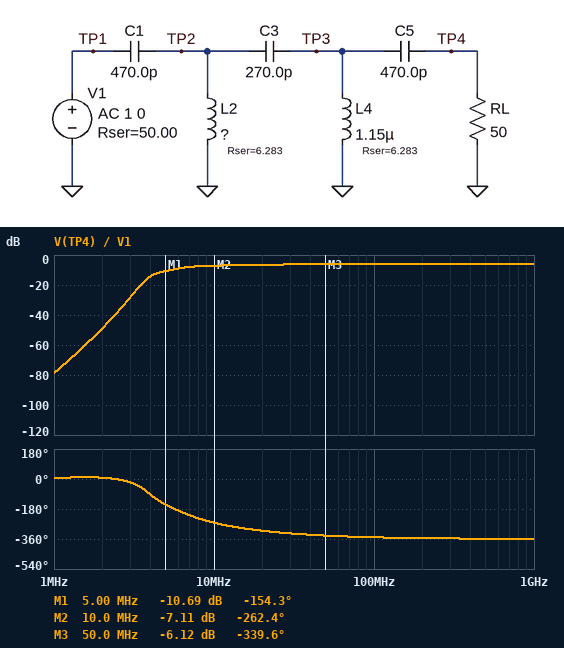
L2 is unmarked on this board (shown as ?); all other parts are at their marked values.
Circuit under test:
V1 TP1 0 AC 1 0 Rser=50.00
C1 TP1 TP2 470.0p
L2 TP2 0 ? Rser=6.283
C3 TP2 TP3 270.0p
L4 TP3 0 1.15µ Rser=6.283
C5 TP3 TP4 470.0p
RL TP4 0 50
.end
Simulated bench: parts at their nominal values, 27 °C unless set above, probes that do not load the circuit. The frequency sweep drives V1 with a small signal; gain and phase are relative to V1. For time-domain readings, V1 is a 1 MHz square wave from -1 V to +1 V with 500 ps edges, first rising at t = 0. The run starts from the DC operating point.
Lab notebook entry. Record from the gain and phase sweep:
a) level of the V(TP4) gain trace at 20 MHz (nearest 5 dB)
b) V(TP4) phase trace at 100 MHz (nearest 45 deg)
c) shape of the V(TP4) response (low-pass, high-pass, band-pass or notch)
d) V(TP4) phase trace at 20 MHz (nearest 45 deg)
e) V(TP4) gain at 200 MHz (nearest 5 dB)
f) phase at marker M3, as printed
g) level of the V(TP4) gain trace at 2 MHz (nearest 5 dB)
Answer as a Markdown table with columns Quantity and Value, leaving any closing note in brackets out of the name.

| Quantity | Value |
|---|---|
| level of the V(TP4) gain trace at 20 MHz | -5 dB |
| V(TP4) phase trace at 100 MHz | -360 deg |
| shape of the V(TP4) response | high-pass |
| V(TP4) phase trace at 20 MHz | -315 deg |
| V(TP4) gain at 200 MHz | -5 dB |
| phase at marker M3, as printed | -339.6 deg |
| level of the V(TP4) gain trace at 2 MHz | -50 dB |
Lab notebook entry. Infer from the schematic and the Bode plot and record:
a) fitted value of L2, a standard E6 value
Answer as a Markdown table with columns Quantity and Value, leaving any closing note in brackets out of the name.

| Quantity | Value |
|---|---|
| fitted value of L2, a standard E6 value | 2.2 µH |
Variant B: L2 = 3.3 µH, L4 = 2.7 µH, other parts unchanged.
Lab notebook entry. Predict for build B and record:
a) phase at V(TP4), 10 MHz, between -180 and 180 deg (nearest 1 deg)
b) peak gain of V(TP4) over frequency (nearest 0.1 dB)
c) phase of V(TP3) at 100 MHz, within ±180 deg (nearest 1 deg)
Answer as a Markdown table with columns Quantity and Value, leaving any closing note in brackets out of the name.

| Quantity | Value |
|---|---|
| phase at V(TP4), 10 MHz, between -180 and 180 deg | 73 deg |
| peak gain of V(TP4) over frequency | -6.0 dB |
| phase of V(TP3) at 100 MHz, within ±180 deg | 5 deg |
